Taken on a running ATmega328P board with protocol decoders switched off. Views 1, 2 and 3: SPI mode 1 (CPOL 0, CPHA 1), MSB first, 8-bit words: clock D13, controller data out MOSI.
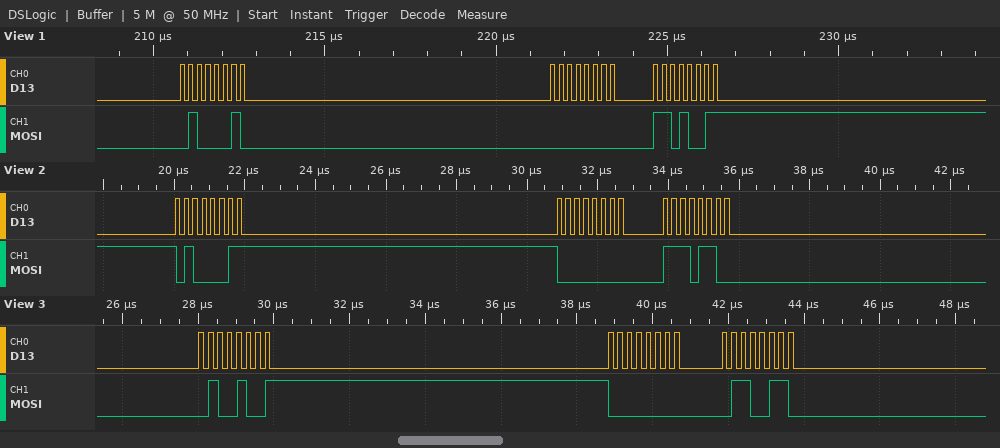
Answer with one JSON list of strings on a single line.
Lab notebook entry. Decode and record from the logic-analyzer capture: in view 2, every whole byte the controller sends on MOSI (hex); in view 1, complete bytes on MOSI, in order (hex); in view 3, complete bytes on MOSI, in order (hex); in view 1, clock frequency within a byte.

["43 00 EC", "42 00 D3", "49 00 66", "4 MHz"]
